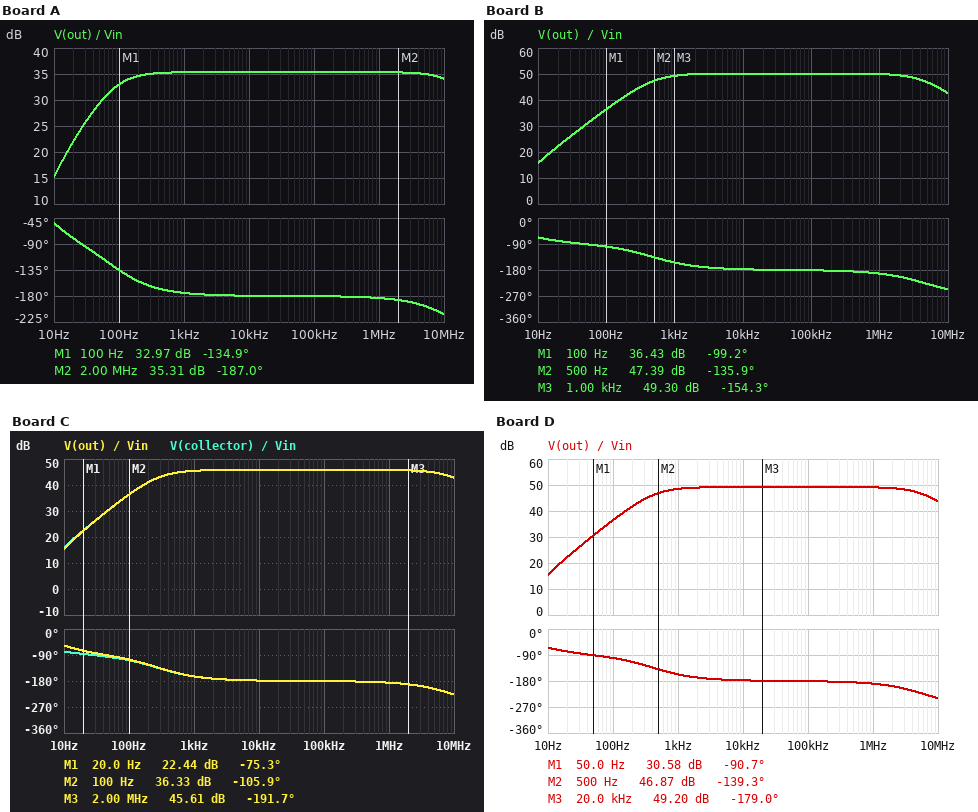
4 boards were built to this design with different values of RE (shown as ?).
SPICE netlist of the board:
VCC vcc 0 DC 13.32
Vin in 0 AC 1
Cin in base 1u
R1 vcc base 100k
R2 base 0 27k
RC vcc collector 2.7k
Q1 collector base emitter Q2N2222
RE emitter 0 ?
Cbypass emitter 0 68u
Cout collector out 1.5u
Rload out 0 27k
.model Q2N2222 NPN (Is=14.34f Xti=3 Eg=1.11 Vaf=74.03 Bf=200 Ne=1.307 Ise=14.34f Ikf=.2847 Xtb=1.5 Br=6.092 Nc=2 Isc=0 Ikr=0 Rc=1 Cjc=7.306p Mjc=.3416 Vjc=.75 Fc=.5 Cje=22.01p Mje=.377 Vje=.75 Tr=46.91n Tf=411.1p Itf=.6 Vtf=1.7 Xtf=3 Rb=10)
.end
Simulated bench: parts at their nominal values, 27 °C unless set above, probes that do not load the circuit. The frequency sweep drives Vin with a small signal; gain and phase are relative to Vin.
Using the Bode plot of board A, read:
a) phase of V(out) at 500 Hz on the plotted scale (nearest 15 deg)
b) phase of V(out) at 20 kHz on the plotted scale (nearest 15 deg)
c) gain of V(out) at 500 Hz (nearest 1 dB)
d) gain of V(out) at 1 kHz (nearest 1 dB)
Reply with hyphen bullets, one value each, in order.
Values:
- -165 deg
- -180 deg
- 35 dB
- 35 dB
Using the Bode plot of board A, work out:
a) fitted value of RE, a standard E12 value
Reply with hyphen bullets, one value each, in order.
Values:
- 3.3 kΩ
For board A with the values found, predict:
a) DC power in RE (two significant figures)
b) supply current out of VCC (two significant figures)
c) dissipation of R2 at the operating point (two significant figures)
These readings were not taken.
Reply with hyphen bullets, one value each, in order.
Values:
- 1.3 mW
- 740 µA
- 280 µW
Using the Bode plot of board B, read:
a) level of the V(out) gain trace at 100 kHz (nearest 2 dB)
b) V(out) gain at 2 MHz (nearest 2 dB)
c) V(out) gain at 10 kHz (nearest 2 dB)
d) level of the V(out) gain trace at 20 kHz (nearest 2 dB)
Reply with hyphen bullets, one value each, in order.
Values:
- 50 dB
- 50 dB
- 50 dB
- 50 dB
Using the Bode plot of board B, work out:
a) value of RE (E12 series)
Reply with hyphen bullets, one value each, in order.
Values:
- 390 Ω
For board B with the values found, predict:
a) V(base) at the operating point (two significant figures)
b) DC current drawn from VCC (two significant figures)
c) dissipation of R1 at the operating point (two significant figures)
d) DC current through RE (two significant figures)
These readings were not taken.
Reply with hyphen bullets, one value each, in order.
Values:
- 2.2 V
- 4.1 mA
- 1.2 mW
- 4.0 mA
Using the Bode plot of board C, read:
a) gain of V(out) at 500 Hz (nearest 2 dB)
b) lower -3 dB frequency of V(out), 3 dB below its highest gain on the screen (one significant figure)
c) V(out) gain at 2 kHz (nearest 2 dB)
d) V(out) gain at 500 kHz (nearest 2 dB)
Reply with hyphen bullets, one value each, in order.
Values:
- 44 dB
- 300 Hz
- 46 dB
- 46 dB
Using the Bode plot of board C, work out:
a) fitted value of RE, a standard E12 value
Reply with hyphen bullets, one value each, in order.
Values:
- 820 Ω
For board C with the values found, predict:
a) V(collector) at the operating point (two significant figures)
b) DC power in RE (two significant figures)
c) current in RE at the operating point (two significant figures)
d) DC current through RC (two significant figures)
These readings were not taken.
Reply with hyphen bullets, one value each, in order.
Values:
- 7.3 V
- 4.1 mW
- 2.2 mA
- 2.2 mA
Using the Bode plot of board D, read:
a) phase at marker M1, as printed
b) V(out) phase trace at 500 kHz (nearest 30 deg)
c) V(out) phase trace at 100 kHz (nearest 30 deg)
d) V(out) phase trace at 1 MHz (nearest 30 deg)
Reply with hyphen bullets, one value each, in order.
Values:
- -90.7 deg
- -180 deg
- -180 deg
- -180 deg
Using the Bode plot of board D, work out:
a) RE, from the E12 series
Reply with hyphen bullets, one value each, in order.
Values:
- 470 Ω
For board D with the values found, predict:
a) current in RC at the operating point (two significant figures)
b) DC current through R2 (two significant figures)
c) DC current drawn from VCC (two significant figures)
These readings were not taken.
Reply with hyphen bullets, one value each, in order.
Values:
- 3.5 mA
- 86 µA
- 3.6 mA
